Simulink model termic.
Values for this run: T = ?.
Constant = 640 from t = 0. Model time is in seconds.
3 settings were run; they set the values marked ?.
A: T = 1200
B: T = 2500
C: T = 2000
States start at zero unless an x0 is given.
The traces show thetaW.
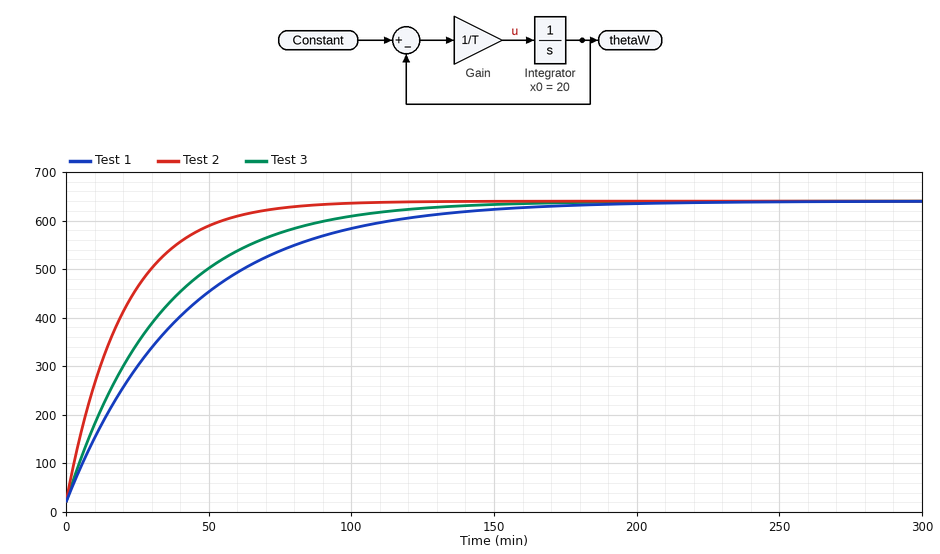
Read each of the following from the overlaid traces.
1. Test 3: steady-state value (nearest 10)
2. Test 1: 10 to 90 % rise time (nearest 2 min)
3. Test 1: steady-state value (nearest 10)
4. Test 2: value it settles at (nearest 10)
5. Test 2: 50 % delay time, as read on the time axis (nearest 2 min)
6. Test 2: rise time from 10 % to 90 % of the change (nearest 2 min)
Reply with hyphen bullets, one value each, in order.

- 640
- 92 min
- 640
- 640
- 14 min
- 44 min
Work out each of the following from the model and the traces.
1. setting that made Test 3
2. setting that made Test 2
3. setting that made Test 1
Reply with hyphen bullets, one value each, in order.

- C
- A
- B
